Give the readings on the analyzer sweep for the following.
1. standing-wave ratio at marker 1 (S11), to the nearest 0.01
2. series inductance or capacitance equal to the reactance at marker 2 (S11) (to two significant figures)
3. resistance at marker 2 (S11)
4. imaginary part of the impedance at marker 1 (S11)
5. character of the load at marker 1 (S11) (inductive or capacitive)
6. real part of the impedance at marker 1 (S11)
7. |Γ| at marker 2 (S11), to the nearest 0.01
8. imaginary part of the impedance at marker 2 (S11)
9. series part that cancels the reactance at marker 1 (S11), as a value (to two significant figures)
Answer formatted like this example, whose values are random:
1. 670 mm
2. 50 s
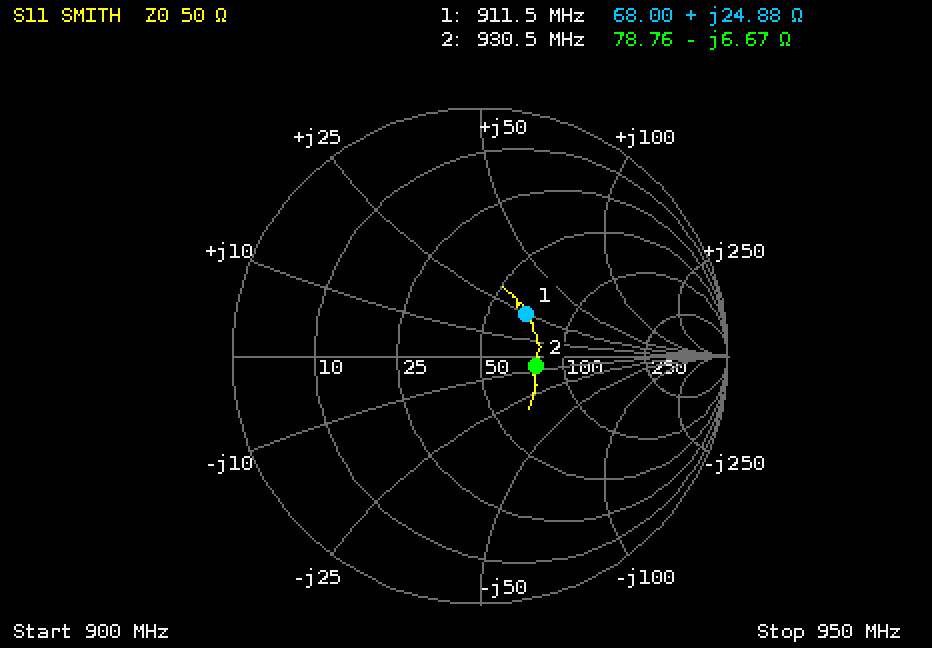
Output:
1. 1.68
2. 26 pF
3. 78.76 Ω
4. +24.88 Ω
5. inductive
6. 68.00 Ω
7. 0.23
8. -6.67 Ω
9. 7.0 pF
